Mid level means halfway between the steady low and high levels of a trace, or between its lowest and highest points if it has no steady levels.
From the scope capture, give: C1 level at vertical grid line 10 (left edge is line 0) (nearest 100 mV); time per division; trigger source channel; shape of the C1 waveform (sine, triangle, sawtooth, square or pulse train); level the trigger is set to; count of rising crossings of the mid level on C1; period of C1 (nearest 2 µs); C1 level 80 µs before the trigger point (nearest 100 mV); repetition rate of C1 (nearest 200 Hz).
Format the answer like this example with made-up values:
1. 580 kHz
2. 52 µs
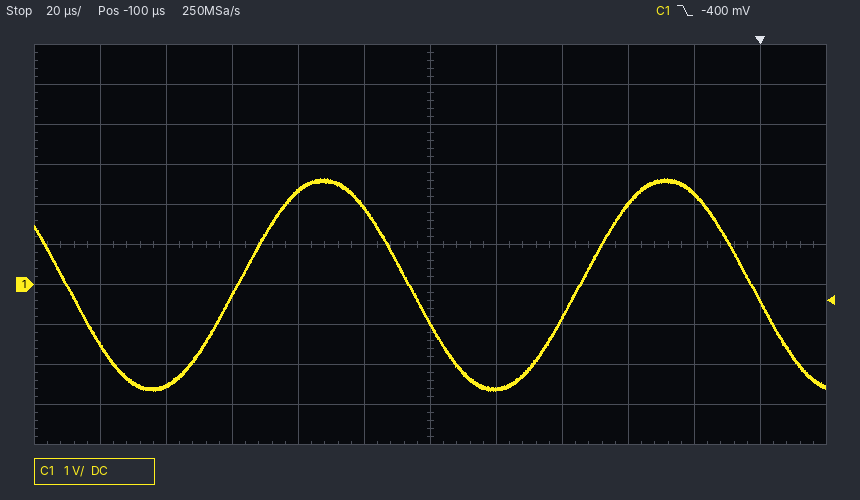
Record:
1. 2.3 V
2. 20 µs
3. C1
4. sine
5. -400 mV
6. 2
7. 104 µs
8. -2.6 V
9. 9.6 kHz
